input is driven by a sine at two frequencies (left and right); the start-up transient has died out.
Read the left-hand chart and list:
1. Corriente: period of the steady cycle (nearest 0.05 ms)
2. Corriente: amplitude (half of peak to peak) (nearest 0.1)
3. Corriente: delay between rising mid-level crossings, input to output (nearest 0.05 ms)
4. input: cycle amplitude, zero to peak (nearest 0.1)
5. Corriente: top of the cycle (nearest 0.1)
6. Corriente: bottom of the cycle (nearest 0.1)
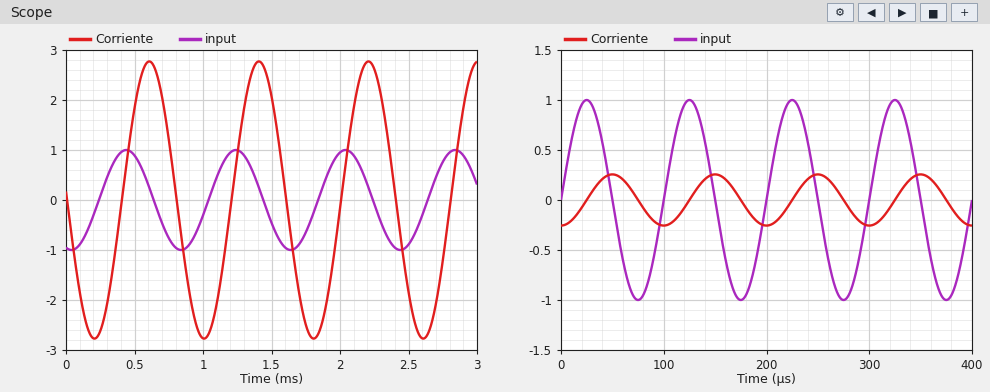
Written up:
0.80 ms
2.8
0.15 ms
1.0
2.8
-2.8
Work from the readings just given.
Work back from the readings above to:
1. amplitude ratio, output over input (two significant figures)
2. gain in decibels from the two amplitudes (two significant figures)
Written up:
2.8
8.9 dB
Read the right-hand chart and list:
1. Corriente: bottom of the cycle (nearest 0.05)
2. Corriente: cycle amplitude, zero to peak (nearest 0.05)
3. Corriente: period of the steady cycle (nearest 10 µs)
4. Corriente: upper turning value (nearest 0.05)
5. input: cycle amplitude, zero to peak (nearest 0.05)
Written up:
-0.25
0.25
100 µs
0.25
1.00
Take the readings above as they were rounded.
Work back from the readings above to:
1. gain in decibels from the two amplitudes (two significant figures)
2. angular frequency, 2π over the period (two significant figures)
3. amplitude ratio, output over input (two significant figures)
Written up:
-12 dB
0.063 rad/µs
0.25
